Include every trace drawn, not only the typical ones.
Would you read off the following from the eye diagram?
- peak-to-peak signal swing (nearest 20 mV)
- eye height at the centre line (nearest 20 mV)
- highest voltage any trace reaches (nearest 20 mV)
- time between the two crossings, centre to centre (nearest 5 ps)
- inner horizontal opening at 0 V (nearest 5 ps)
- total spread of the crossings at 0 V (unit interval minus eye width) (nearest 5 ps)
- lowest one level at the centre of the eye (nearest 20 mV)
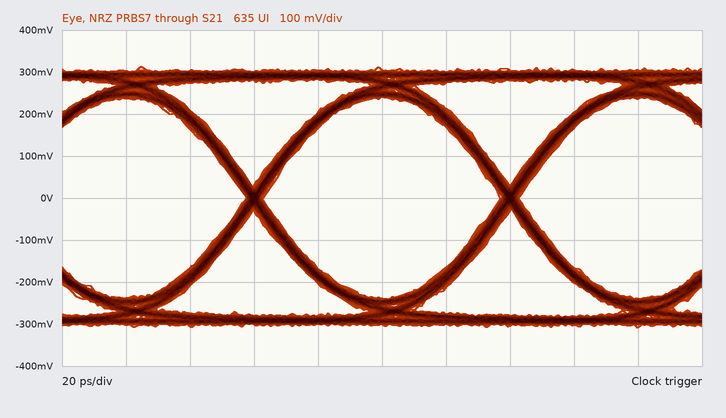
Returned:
620 mV
480 mV
320 mV
80 ps
75 ps
5 ps
240 mV
